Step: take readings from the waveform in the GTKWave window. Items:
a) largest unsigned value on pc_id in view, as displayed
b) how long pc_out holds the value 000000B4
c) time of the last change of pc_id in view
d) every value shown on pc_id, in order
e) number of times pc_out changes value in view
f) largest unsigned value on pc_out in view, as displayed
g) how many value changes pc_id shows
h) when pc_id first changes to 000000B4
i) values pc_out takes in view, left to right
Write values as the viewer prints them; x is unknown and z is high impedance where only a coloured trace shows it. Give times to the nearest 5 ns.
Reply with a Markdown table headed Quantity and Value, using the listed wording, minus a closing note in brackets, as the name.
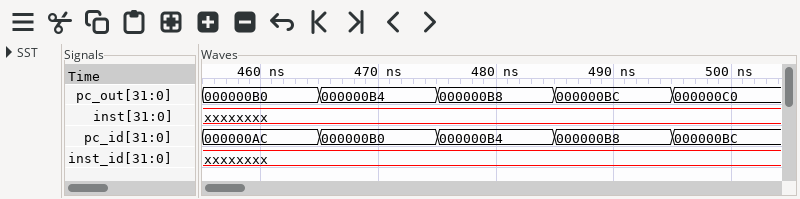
| Quantity | Value |
|---|---|
| largest unsigned value on pc_id in view, as displayed | 000000BC |
| how long pc_out holds the value 000000B4 | 10 ns |
| time of the last change of pc_id in view | 495 ns |
| every value shown on pc_id, in order | 000000AC, 000000B0, 000000B4, 000000B8, 000000BC |
| number of times pc_out changes value in view | 4 |
| largest unsigned value on pc_out in view, as displayed | 000000C0 |
| how many value changes pc_id shows | 4 |
| when pc_id first changes to 000000B4 | 475 ns |
| values pc_out takes in view, left to right | 000000B0, 000000B4, 000000B8, 000000BC, 000000C0 |
